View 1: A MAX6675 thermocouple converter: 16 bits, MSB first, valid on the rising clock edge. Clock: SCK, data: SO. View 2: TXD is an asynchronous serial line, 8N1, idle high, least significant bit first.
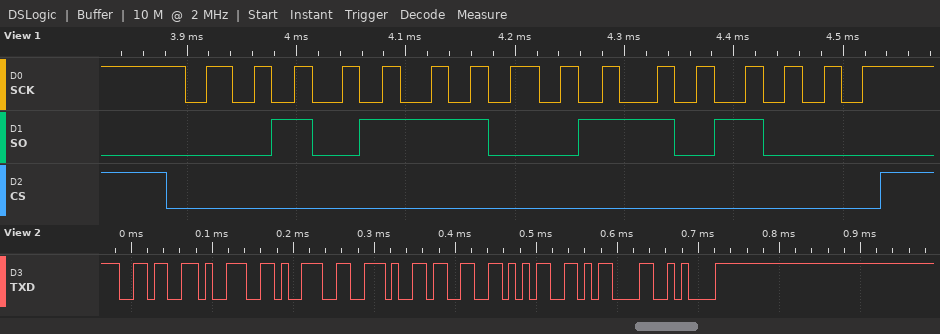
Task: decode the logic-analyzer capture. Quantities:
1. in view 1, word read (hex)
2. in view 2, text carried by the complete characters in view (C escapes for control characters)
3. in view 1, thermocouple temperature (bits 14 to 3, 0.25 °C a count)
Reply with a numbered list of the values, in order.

1. 0x2E68
2. "699.35\r\n"
3. 371.25 °C
